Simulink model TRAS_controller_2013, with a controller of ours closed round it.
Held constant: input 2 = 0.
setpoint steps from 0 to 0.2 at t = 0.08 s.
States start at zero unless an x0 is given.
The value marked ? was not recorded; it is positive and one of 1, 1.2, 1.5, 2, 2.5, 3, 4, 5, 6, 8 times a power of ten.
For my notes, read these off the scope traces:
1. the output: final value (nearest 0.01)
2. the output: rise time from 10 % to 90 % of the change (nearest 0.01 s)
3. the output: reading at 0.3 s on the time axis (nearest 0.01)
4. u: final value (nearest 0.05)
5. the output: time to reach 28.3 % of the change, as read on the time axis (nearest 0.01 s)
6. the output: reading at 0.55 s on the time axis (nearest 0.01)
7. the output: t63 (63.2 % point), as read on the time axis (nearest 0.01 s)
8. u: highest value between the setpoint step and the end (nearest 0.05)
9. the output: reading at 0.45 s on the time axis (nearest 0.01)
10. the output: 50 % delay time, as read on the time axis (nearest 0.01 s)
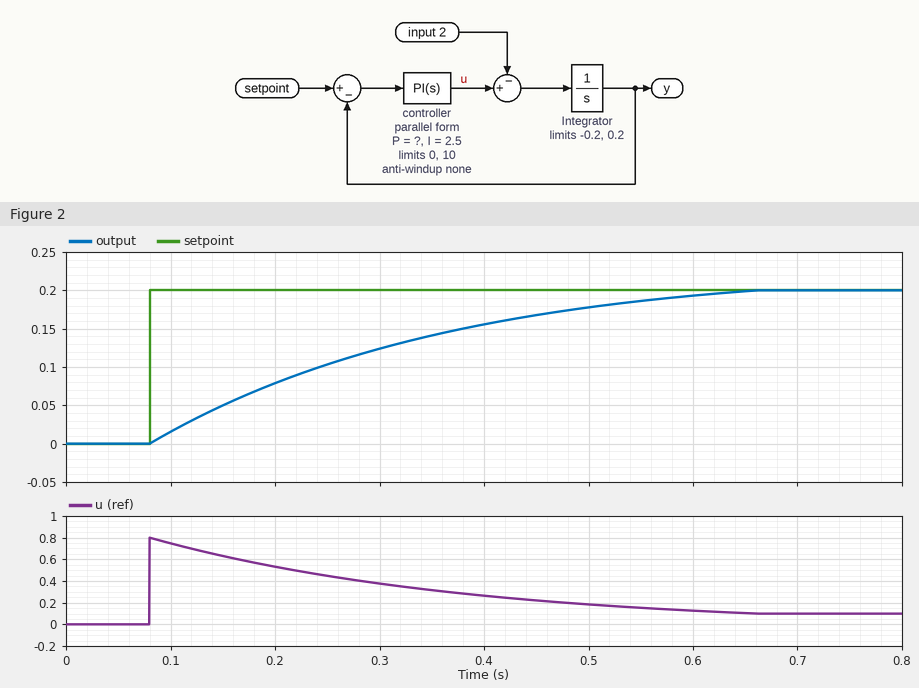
0.20
0.41 s
0.12
0.10
0.16 s
0.19
0.31 s
0.80
0.17
0.24 s
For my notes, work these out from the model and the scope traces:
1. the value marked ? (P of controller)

4
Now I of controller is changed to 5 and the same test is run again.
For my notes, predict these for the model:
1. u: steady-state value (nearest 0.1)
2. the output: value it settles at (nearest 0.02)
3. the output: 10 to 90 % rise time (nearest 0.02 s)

0.2
0.20
0.34 s
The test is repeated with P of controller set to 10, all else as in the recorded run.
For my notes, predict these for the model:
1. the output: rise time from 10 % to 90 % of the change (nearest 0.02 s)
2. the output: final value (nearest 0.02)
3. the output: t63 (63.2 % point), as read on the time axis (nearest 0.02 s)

0.20 s
0.20
0.18 s
